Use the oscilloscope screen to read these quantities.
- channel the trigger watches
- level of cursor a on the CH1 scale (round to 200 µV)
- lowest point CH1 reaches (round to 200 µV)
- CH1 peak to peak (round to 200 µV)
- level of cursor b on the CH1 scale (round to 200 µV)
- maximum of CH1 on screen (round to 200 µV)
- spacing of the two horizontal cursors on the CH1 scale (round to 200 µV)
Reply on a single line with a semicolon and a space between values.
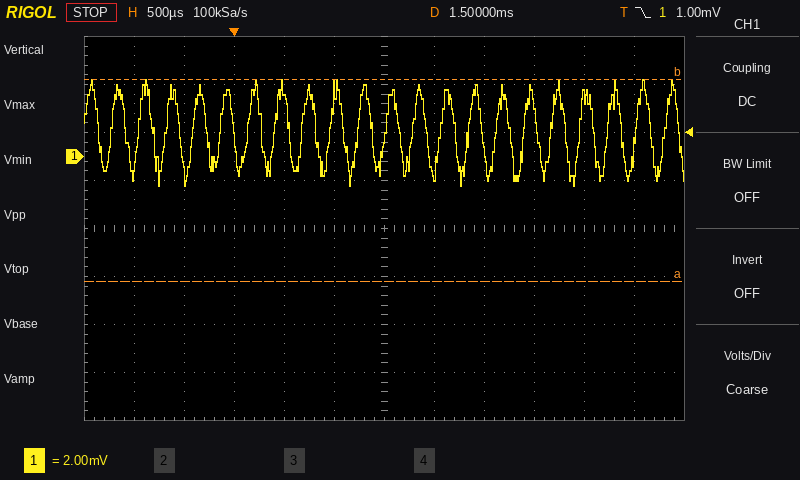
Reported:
CH1; -5.2 mV; -1.2 mV; 4.4 mV; 3.2 mV; 3.2 mV; 8.4 mV
